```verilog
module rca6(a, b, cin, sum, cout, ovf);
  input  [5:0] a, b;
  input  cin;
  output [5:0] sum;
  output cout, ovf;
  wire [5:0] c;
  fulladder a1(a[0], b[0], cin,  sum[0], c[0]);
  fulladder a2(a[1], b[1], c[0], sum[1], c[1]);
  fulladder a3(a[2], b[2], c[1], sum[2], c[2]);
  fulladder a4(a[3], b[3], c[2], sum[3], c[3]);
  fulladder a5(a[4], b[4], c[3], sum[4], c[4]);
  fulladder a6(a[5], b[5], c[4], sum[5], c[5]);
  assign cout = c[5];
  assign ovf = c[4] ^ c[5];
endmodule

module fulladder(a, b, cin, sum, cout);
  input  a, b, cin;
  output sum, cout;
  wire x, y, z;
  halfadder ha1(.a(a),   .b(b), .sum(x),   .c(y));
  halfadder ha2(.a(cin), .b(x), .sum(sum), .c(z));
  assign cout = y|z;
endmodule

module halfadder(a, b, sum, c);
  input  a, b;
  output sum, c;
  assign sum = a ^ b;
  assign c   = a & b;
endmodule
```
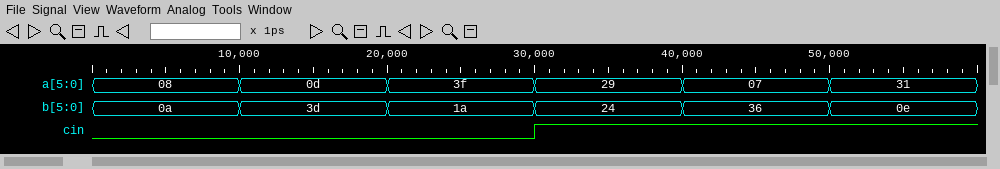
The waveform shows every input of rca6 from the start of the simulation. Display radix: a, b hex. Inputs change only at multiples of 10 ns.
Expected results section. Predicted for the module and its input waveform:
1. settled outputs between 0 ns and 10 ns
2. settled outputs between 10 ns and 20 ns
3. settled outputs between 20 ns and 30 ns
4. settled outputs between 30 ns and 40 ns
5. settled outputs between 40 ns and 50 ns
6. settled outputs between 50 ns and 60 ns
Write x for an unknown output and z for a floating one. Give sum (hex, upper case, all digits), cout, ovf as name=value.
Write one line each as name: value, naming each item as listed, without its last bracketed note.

settled outputs between 0 ns and 10 ns: sum=12, cout=0, ovf=0
settled outputs between 10 ns and 20 ns: sum=0A, cout=1, ovf=0
settled outputs between 20 ns and 30 ns: sum=19, cout=1, ovf=0
settled outputs between 30 ns and 40 ns: sum=0E, cout=1, ovf=1
settled outputs between 40 ns and 50 ns: sum=3E, cout=0, ovf=0
settled outputs between 50 ns and 60 ns: sum=00, cout=1, ovf=0
